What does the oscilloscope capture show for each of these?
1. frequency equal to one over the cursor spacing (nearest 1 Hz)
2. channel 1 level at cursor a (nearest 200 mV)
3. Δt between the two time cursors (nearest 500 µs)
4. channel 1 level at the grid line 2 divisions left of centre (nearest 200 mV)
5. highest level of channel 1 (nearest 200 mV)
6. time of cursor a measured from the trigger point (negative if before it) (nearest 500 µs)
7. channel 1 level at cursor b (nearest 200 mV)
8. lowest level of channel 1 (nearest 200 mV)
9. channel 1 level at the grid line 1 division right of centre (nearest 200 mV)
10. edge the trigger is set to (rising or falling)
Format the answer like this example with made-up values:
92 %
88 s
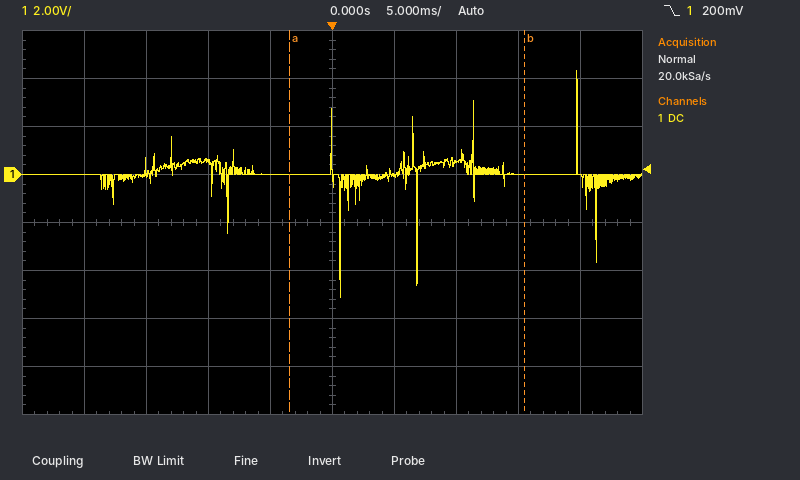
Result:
53 Hz
0.0 V
19.0 ms
600 mV
4.4 V
-3.5 ms
0.0 V
-5.2 V
0.0 V
falling
